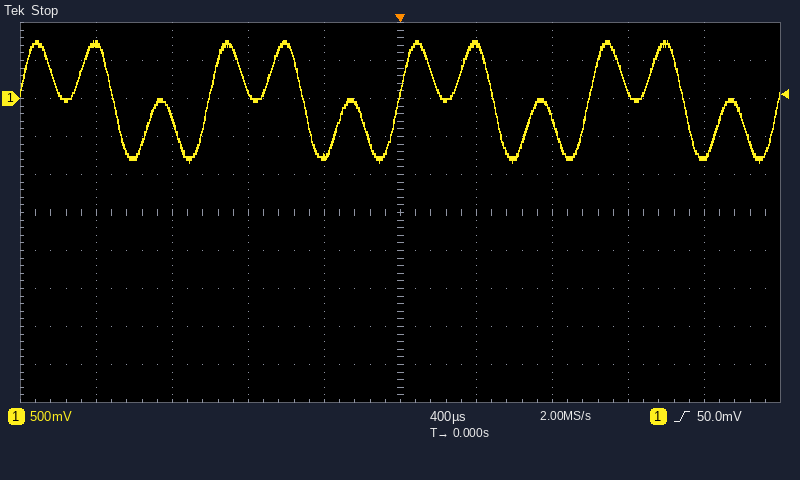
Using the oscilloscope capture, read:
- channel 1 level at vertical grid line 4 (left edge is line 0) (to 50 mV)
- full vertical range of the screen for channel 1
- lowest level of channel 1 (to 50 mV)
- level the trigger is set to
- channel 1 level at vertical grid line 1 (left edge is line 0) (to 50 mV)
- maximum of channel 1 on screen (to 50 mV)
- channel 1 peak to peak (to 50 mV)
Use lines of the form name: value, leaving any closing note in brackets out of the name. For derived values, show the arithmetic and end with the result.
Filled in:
channel 1 level at vertical grid line 4 (left edge is line 0): -750 mV
full vertical range of the screen for channel 1: 5 V
lowest level of channel 1: -850 mV
level the trigger is set to: 50.0 mV
channel 1 level at vertical grid line 1 (left edge is line 0): 700 mV
maximum of channel 1 on screen: 750 mV
channel 1 peak to peak: 750 mV − (-850 mV) = 1.60 V
